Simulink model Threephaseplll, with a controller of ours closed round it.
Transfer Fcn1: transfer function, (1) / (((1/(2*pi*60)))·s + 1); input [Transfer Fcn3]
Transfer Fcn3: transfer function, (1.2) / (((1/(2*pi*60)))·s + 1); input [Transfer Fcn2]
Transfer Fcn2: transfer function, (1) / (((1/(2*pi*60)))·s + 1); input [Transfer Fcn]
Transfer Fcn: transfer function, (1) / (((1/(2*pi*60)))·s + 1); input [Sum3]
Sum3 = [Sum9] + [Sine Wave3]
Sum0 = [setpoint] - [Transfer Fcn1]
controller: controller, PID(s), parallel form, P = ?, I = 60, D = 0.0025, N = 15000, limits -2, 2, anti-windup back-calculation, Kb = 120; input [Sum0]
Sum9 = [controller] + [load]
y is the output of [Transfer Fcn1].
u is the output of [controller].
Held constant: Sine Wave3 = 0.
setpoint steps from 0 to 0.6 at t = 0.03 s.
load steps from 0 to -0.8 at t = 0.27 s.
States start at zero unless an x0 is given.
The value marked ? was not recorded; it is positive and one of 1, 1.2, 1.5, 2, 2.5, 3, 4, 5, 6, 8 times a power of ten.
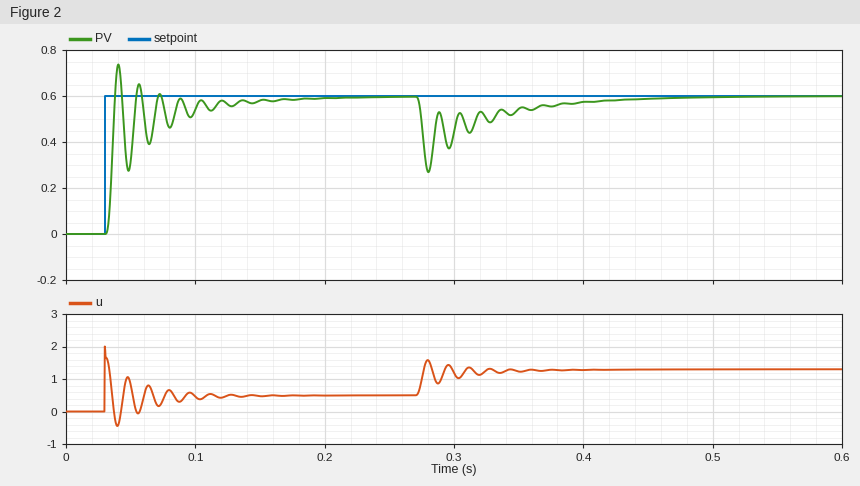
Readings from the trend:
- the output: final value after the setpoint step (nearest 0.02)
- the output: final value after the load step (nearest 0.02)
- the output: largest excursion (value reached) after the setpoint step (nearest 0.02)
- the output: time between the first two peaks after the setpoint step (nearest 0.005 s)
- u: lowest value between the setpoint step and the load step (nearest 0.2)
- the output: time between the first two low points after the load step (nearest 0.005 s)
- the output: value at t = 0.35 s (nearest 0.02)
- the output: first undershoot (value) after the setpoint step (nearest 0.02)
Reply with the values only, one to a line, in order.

0.60
0.60
0.74
0.015 s
-0.4
0.015 s
0.54
0.28
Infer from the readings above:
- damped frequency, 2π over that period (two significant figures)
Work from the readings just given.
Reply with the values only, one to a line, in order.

420 rad/s
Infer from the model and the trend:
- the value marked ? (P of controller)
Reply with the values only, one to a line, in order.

3
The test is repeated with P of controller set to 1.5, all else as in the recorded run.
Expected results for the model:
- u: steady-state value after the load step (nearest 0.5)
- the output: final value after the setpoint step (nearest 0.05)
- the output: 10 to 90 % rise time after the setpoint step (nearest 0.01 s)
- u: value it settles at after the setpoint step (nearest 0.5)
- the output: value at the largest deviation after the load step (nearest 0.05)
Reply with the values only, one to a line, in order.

1.5
0.60
0.05 s
0.5
0.20
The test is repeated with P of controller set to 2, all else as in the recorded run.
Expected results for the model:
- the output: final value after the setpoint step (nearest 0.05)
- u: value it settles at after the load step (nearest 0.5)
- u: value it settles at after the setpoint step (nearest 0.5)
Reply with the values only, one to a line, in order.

0.60
1.5
0.5
